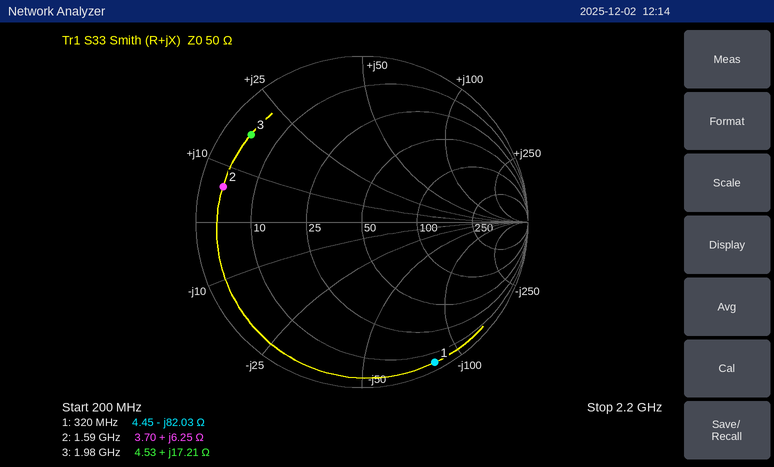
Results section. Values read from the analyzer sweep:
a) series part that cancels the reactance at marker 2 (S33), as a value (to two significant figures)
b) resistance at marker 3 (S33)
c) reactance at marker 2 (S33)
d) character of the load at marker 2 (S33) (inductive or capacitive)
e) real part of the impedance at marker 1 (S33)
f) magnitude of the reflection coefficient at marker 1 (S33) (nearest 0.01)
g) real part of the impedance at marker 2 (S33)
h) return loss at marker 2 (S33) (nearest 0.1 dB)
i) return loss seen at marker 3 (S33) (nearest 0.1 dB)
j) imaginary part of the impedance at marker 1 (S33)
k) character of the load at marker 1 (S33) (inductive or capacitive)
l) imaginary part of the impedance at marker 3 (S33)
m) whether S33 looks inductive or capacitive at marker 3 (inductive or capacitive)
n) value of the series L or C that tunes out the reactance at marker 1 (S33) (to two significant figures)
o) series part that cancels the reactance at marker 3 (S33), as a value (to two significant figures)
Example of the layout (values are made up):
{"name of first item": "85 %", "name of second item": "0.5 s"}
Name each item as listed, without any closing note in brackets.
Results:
{"series part that cancels the reactance at marker 2 (S33), as a value": "16 pF", "resistance at marker 3": "4.53 Ω", "reactance at marker 2": "+6.25 Ω", "character of the load at marker 2 (S33)": "inductive", "real part of the impedance at marker 1": "4.45 Ω", "magnitude of the reflection coefficient at marker 1 (S33)": "0.95", "real part of the impedance at marker 2": "3.70 Ω", "return loss at marker 2 (S33)": "1.3 dB", "return loss seen at marker 3 (S33)": "1.4 dB", "imaginary part of the impedance at marker 1": "-82.03 Ω", "character of the load at marker 1 (S33)": "capacitive", "imaginary part of the impedance at marker 3": "+17.21 Ω", "whether S33 looks inductive or capacitive at marker 3": "inductive", "value of the series L or C that tunes out the reactance at marker 1 (S33)": "41 nH", "series part that cancels the reactance at marker 3 (S33), as a value": "4.7 pF"}
